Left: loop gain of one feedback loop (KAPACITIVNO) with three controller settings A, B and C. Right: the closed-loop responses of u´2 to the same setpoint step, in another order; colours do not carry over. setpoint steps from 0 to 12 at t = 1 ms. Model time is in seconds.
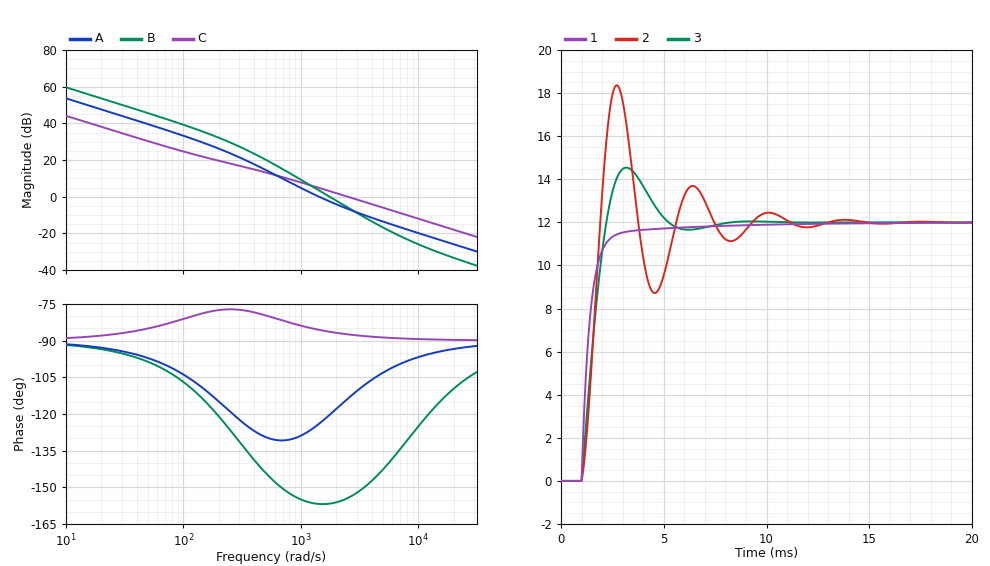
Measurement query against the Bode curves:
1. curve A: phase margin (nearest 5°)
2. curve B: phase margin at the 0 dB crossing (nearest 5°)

55°
25°
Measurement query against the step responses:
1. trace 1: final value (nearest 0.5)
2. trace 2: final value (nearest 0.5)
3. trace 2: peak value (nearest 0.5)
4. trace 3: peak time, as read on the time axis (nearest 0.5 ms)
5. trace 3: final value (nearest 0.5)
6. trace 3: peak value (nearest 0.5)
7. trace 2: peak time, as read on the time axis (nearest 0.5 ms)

12.0
12.0
18.5
3.0 ms
12.0
14.5
2.5 ms
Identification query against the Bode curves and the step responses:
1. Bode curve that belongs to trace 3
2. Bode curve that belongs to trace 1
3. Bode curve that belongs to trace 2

A
C
B
